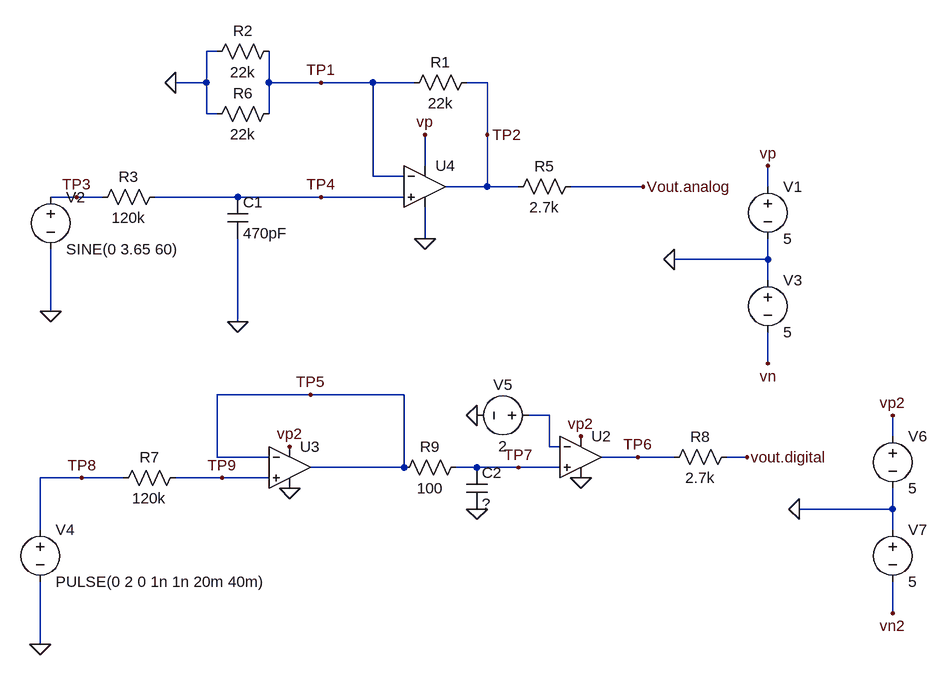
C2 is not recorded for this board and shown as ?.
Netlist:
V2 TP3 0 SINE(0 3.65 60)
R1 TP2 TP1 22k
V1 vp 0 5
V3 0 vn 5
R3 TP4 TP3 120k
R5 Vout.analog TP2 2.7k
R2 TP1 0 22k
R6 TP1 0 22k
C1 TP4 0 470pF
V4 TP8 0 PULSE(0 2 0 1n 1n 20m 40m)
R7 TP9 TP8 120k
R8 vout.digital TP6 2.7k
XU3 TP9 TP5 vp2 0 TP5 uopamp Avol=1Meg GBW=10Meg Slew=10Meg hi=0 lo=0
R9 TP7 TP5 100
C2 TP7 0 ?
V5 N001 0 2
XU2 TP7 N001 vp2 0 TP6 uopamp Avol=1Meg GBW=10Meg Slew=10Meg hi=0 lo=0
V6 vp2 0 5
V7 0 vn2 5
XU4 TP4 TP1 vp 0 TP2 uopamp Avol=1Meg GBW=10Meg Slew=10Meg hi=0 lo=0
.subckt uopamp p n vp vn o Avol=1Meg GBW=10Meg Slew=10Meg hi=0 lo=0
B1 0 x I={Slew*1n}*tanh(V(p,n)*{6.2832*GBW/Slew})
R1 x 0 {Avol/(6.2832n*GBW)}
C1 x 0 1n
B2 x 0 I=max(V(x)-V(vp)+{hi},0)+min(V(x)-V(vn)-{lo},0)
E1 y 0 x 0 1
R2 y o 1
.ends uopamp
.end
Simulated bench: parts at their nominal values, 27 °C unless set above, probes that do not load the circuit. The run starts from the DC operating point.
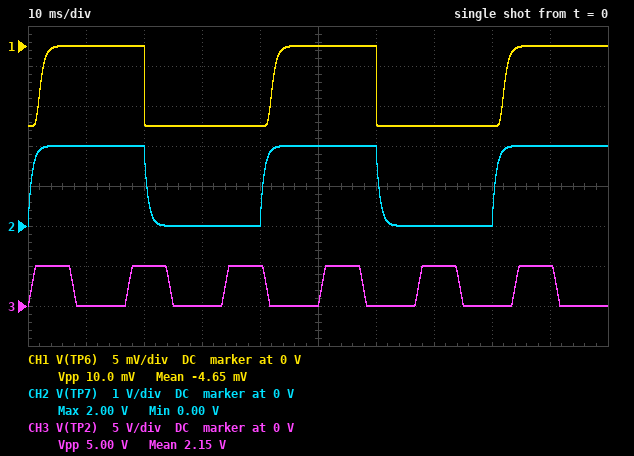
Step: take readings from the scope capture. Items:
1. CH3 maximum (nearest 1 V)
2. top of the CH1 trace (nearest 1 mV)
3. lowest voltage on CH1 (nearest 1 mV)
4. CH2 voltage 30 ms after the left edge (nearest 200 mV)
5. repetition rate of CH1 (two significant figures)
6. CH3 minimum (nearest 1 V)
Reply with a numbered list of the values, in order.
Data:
1. 5 V
2. 0 V
3. -10 mV
4. 0 V
5. 25 Hz
6. 0 V
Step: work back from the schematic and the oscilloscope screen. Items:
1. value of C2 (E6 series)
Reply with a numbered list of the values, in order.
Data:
1. 6.8 µF
